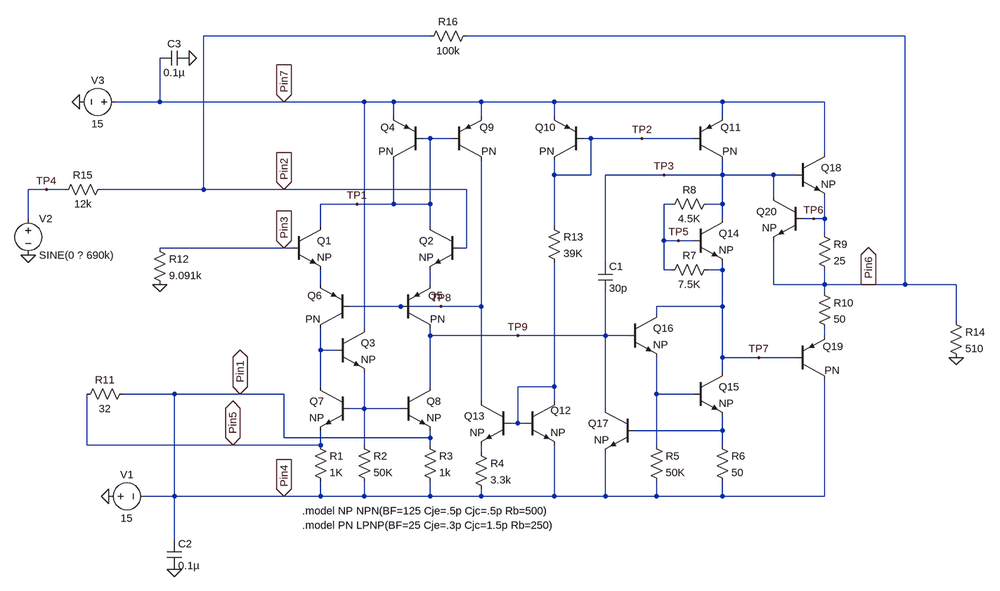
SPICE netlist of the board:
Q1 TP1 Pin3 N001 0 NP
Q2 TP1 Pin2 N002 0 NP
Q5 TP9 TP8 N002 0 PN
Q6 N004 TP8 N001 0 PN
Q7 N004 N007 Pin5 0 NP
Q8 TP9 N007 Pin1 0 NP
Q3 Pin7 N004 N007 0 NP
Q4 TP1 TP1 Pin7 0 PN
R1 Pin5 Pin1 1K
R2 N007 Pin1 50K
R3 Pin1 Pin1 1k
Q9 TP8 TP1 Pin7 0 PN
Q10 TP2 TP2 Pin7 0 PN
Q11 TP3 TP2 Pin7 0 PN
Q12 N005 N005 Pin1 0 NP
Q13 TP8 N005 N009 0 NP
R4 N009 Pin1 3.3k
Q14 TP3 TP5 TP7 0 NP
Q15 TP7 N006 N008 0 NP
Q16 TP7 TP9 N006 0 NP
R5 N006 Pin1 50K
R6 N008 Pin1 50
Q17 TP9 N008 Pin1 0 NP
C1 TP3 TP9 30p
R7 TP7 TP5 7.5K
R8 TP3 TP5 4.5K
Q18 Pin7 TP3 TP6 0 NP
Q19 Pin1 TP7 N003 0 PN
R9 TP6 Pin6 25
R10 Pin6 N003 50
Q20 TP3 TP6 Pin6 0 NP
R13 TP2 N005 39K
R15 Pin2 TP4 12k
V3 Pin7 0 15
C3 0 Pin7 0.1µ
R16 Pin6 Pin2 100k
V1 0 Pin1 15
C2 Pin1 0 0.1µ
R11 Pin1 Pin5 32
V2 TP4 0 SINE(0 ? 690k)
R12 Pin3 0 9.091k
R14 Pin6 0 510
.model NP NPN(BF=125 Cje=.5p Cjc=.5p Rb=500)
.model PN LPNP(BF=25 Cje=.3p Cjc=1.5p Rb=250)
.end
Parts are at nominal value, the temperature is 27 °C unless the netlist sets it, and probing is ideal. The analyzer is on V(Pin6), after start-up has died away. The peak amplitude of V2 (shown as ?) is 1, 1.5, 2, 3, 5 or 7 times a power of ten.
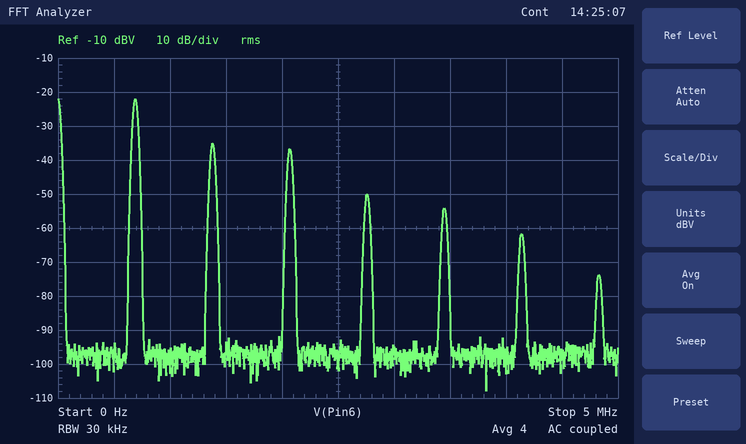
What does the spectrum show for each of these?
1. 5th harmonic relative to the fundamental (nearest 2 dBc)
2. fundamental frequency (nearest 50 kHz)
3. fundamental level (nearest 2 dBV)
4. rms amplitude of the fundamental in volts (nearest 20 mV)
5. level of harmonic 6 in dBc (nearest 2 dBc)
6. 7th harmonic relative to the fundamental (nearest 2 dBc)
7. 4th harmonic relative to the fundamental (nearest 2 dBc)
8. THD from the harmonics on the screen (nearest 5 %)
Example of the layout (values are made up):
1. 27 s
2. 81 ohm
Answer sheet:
1. -32 dBc
2. 700 kHz
3. -22 dBV
4. 80 mV
5. -40 dBc
6. -52 dBc
7. -28 dBc
8. 30 %
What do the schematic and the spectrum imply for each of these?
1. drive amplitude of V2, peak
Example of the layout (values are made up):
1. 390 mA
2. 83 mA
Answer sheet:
1. 300 mV
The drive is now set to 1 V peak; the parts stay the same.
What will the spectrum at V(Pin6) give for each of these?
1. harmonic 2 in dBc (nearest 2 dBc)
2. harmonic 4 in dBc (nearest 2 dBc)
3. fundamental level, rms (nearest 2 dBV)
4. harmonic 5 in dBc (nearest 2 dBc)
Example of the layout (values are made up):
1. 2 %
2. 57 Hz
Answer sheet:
1. -18 dBc
2. -26 dBc
3. -22 dBV
4. -24 dBc
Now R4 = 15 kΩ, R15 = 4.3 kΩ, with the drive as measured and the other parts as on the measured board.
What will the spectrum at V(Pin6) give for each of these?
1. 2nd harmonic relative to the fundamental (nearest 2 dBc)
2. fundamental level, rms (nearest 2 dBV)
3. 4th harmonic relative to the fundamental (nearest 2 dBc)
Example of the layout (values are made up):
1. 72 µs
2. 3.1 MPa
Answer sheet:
1. -26 dBc
2. -32 dBV
3. -34 dBc
